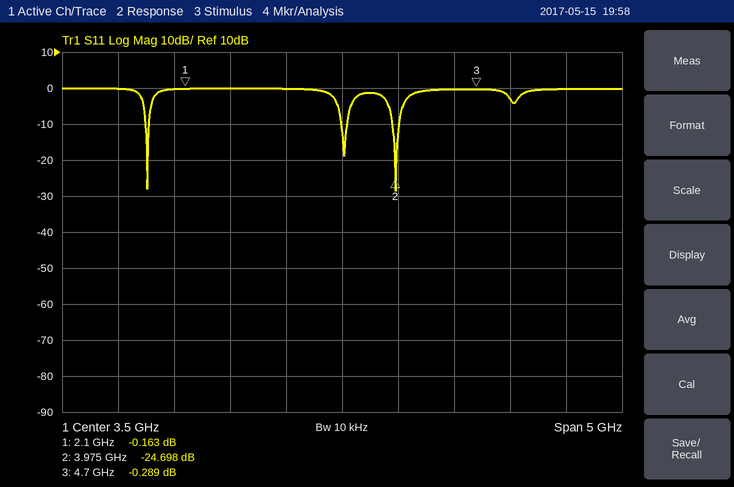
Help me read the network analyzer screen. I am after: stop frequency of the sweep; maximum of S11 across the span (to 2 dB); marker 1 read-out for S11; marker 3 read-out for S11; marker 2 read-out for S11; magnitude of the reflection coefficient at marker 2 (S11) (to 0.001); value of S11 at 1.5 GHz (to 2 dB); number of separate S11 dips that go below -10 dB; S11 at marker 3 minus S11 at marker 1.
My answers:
6 GHz
0 dB
-0.163 dB
-0.289 dB
-24.698 dB
0.058
0 dB
3
-0.126 dB
